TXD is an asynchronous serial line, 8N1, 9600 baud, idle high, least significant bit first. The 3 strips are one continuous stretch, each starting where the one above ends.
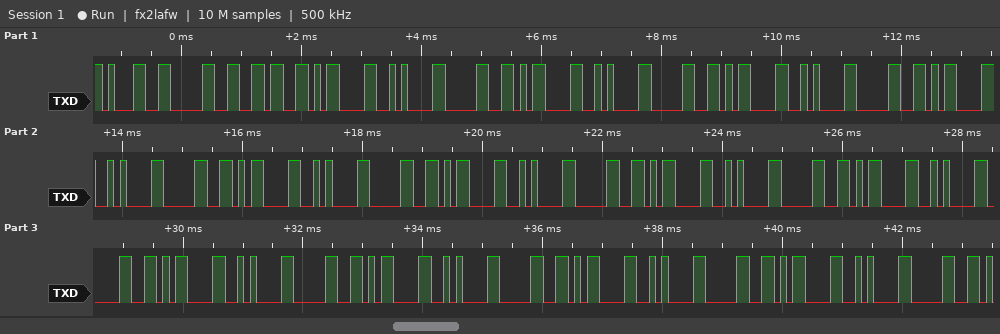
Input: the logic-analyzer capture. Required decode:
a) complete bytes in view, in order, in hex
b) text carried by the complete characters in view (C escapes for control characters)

31 30 36 0D 0A 30 0D 0A 30 0D 0A 30 0D 0A 30 0D 0A 30 0D 0A 30 0D 0A 30 0D 0A 30 0D 0A 30 0D 0A 30 0D 0A 30 0D 0A 30
"106\r\n0\r\n0\r\n0\r\n0\r\n0\r\n0\r\n0\r\n0\r\n0\r\n0\r\n0\r\n0"
